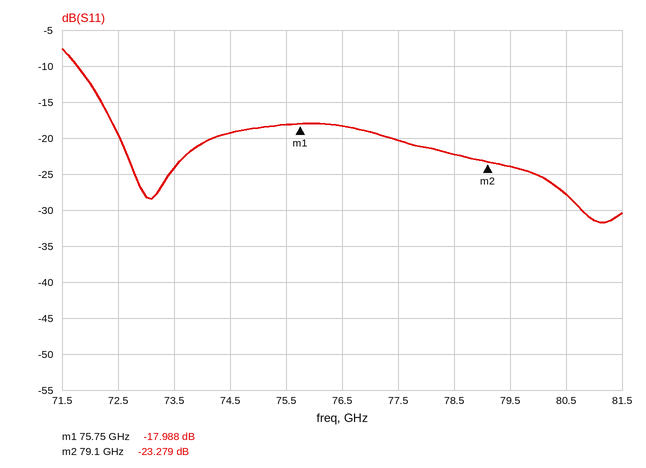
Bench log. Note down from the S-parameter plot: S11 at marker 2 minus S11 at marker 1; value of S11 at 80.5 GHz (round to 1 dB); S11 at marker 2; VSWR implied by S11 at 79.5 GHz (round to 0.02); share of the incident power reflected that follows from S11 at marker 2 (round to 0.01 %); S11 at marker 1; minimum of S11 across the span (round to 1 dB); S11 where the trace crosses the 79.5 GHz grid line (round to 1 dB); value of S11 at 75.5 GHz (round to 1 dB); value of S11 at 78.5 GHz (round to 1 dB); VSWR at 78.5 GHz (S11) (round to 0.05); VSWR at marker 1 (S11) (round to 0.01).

-5.291 dB
-28 dB
-23.279 dB
1.14
0.47 %
-17.988 dB
-32 dB
-24 dB
-18 dB
-22 dB
1.15
1.29
